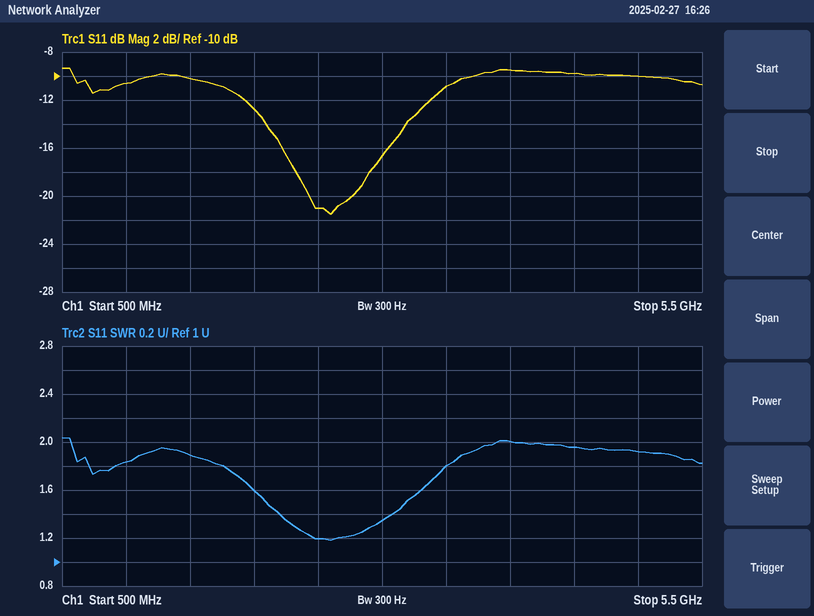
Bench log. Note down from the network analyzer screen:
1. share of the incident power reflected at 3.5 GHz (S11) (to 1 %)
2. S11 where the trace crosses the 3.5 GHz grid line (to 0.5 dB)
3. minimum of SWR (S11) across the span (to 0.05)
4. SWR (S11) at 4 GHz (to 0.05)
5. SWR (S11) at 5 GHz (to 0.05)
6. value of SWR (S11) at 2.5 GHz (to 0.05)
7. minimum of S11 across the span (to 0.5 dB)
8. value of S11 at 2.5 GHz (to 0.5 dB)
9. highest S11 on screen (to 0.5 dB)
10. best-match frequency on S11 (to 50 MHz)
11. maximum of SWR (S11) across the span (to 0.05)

8 %
-11.0 dB
1.20
2.00
1.90
1.20
-21.5 dB
-21.0 dB
-9.5 dB
2.60 GHz
2.05
